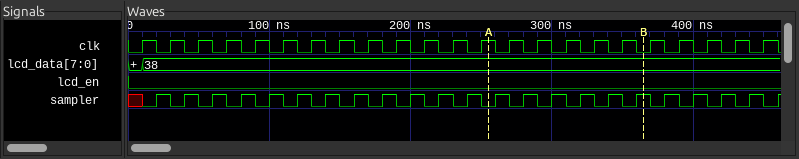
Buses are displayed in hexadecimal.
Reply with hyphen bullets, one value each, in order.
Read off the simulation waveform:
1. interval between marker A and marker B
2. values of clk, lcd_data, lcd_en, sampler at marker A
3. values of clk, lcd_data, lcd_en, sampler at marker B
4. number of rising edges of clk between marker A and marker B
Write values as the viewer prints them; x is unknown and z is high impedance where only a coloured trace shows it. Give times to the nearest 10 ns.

- 110 ns
- clk=1, lcd_data=38, lcd_en=0, sampler=0
- clk=0, lcd_data=38, lcd_en=0, sampler=1
- 5
